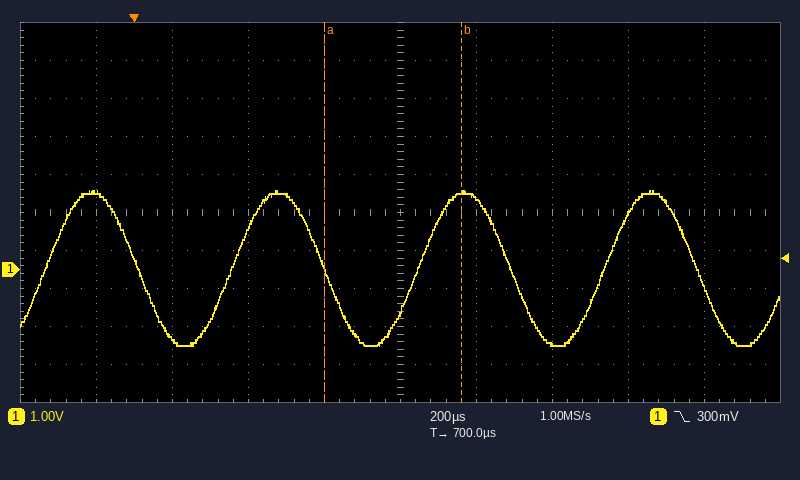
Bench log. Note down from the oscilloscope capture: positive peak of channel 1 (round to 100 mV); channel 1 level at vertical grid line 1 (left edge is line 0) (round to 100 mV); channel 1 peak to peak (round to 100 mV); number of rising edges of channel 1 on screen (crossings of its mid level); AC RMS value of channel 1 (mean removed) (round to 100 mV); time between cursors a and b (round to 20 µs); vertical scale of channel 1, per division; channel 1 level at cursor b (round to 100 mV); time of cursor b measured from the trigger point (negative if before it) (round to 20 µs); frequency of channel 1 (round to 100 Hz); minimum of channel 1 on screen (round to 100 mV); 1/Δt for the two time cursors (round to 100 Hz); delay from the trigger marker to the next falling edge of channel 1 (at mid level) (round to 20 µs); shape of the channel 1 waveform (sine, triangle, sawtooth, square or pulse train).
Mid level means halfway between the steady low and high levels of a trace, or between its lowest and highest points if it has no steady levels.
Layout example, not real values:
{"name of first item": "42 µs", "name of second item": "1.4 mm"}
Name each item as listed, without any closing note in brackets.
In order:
{"positive peak of channel 1": "2.1 V", "channel 1 level at vertical grid line 1 (left edge is line 0)": "2.0 V", "channel 1 peak to peak": "4.1 V", "number of rising edges of channel 1 on screen": "4", "AC RMS value of channel 1 (mean removed)": "1.4 V", "time between cursors a and b": "360 µs", "vertical scale of channel 1, per division": "1 V", "channel 1 level at cursor b": "2.0 V", "time of cursor b measured from the trigger point (negative if before it)": "+860 µs", "frequency of channel 1": "2.0 kHz", "minimum of channel 1 on screen": "-2.0 V", "1/Δt for the two time cursors": "2.8 kHz", "delay from the trigger marker to the next falling edge of channel 1 (at mid level)": "500 µs", "shape of the channel 1 waveform": "sine"}
